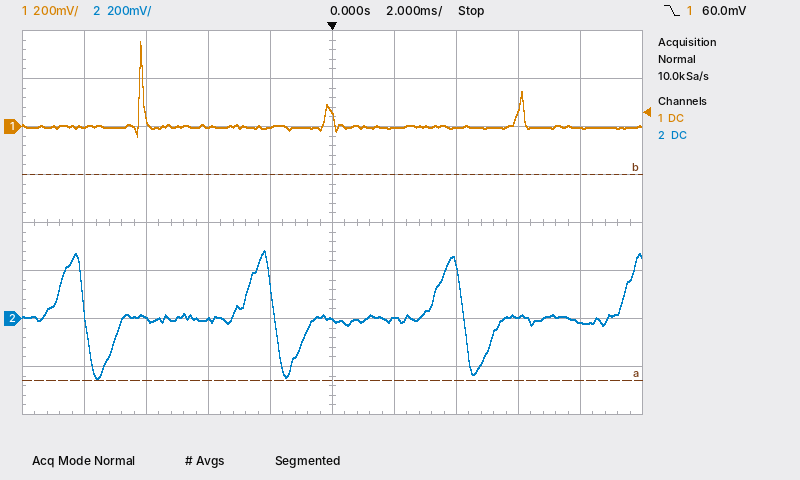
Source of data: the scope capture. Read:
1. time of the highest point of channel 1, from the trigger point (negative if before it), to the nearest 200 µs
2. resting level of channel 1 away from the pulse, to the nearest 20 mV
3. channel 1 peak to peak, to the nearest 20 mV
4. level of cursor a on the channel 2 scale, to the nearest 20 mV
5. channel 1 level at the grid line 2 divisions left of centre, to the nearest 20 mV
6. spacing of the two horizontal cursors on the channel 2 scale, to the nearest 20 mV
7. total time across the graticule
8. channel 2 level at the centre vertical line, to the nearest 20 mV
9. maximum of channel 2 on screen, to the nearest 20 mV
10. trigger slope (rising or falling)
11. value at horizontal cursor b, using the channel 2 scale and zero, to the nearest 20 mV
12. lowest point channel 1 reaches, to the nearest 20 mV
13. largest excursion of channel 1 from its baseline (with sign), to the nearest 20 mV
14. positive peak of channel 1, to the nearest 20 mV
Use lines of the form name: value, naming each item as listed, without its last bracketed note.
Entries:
time of the highest point of channel 1, from the trigger point (negative if before it), to the nearest 200 µs: -6.2 ms
resting level of channel 1 away from the pulse, to the nearest 20 mV: 0 mV
channel 1 peak to peak, to the nearest 20 mV: 400 mV
level of cursor a on the channel 2 scale, to the nearest 20 mV: -260 mV
channel 1 level at the grid line 2 divisions left of centre, to the nearest 20 mV: 0 mV
spacing of the two horizontal cursors on the channel 2 scale, to the nearest 20 mV: 860 mV
total time across the graticule: 20 ms
channel 2 level at the centre vertical line, to the nearest 20 mV: 0 mV
maximum of channel 2 on screen, to the nearest 20 mV: 280 mV
trigger slope: falling
value at horizontal cursor b, using the channel 2 scale and zero, to the nearest 20 mV: 600 mV
lowest point channel 1 reaches, to the nearest 20 mV: -40 mV
largest excursion of channel 1 from its baseline (with sign), to the nearest 20 mV: +360 mV
positive peak of channel 1, to the nearest 20 mV: 360 mV
